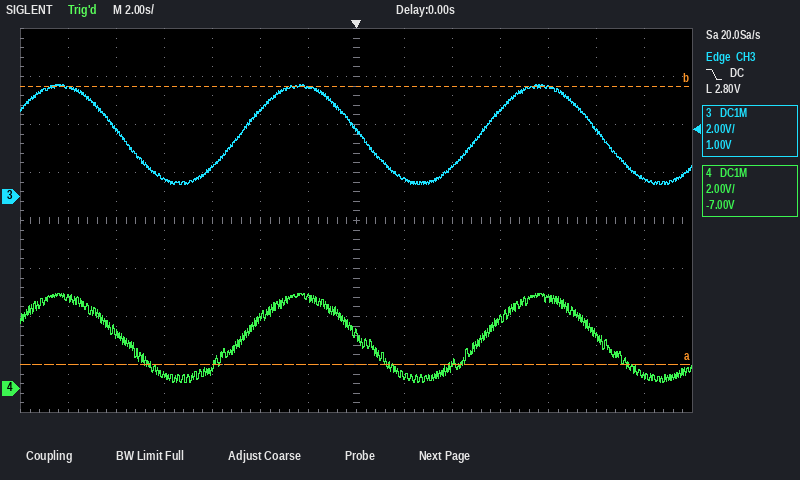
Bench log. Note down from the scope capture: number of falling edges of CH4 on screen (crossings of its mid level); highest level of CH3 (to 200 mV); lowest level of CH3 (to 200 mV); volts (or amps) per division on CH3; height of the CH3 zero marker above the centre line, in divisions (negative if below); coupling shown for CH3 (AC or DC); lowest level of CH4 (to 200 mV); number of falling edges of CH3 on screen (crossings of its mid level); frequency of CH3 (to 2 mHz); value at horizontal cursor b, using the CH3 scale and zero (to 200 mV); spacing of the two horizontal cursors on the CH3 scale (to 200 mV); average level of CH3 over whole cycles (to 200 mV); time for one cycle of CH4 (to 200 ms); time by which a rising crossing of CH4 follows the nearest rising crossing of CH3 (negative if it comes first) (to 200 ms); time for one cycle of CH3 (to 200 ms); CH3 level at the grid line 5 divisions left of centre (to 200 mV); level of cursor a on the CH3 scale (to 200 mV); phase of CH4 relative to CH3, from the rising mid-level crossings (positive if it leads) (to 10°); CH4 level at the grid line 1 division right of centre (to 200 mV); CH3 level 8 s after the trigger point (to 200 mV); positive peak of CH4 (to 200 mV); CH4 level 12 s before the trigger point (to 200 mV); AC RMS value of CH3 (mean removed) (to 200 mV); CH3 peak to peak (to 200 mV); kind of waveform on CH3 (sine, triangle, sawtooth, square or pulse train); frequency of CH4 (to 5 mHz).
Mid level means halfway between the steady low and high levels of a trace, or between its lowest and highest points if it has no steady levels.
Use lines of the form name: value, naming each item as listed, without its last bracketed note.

number of falling edges of CH4 on screen: 3
highest level of CH3: 4.6 V
lowest level of CH3: 400 mV
volts (or amps) per division on CH3: 2 V
height of the CH3 zero marker above the centre line, in divisions: +0.5 div
coupling shown for CH3: DC
lowest level of CH4: 200 mV
number of falling edges of CH3 on screen: 3
frequency of CH3: 100 mHz
value at horizontal cursor b, using the CH3 scale and zero: 4.6 V
spacing of the two horizontal cursors on the CH3 scale: 11.6 V
average level of CH3 over whole cycles: 2.6 V
time for one cycle of CH4: 10.0 s
time by which a rising crossing of CH4 follows the nearest rising crossing of CH3 (negative if it comes first): 0.0 s
time for one cycle of CH3: 10.0 s
CH3 level at the grid line 5 divisions left of centre: 2.8 V
level of cursor a on the CH3 scale: -7.0 V
phase of CH4 relative to CH3, from the rising mid-level crossings (positive if it leads): 0°
CH4 level at the grid line 1 division right of centre: 600 mV
CH3 level 8 s after the trigger point: 4.6 V
positive peak of CH4: 4.0 V
CH4 level 12 s before the trigger point: 3.8 V
AC RMS value of CH3 (mean removed): 1.4 V
CH3 peak to peak: 4.2 V
kind of waveform on CH3: sine
frequency of CH4: 100 mHz
